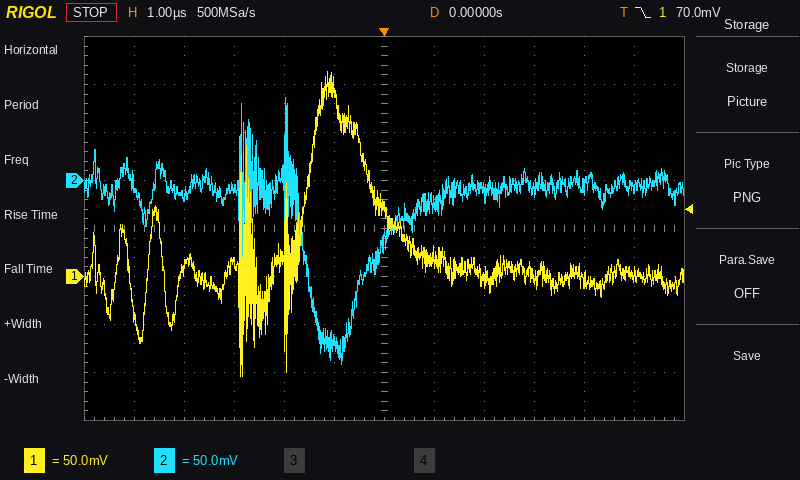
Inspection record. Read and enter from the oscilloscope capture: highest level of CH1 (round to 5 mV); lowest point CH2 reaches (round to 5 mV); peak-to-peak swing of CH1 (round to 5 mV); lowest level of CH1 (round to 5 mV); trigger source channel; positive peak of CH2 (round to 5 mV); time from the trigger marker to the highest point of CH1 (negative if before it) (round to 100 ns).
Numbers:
215 mV
-190 mV
320 mV
-105 mV
CH1
85 mV
-1.1 µs
